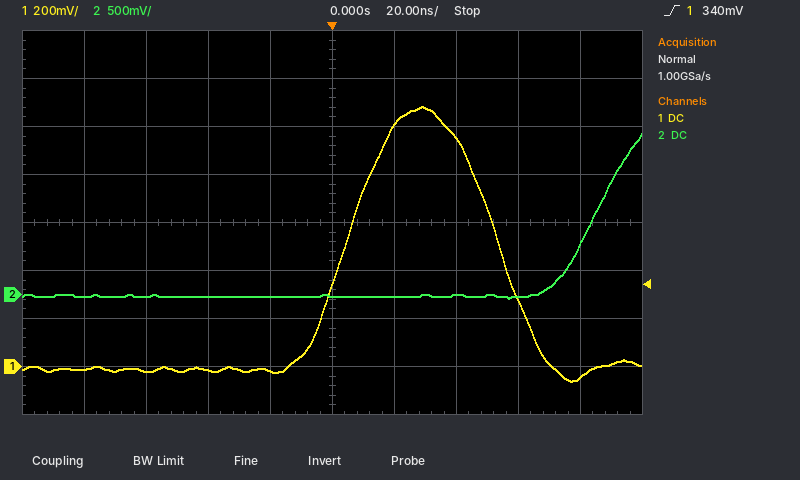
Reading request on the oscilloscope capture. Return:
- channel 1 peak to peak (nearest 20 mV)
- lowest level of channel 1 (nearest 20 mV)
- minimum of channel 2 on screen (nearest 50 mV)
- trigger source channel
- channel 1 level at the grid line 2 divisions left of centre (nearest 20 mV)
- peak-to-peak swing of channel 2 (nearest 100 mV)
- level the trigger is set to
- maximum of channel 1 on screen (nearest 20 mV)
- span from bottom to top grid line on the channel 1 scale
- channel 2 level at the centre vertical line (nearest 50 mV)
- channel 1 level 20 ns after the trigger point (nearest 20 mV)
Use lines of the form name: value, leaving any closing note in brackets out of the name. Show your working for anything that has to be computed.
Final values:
channel 1 peak to peak: 1.08 V − (-60 mV) = 1.14 V
lowest level of channel 1: -60 mV
minimum of channel 2 on screen: -50 mV
trigger source channel: channel 1
channel 1 level at the grid line 2 divisions left of centre: -20 mV
peak-to-peak swing of channel 2: 1.70 V
level the trigger is set to: 340 mV
maximum of channel 1 on screen: 1.08 V
span from bottom to top grid line on the channel 1 scale: 1.6 V
channel 2 level at the centre vertical line: 0 mV
channel 1 level 20 ns after the trigger point: 1.00 V
